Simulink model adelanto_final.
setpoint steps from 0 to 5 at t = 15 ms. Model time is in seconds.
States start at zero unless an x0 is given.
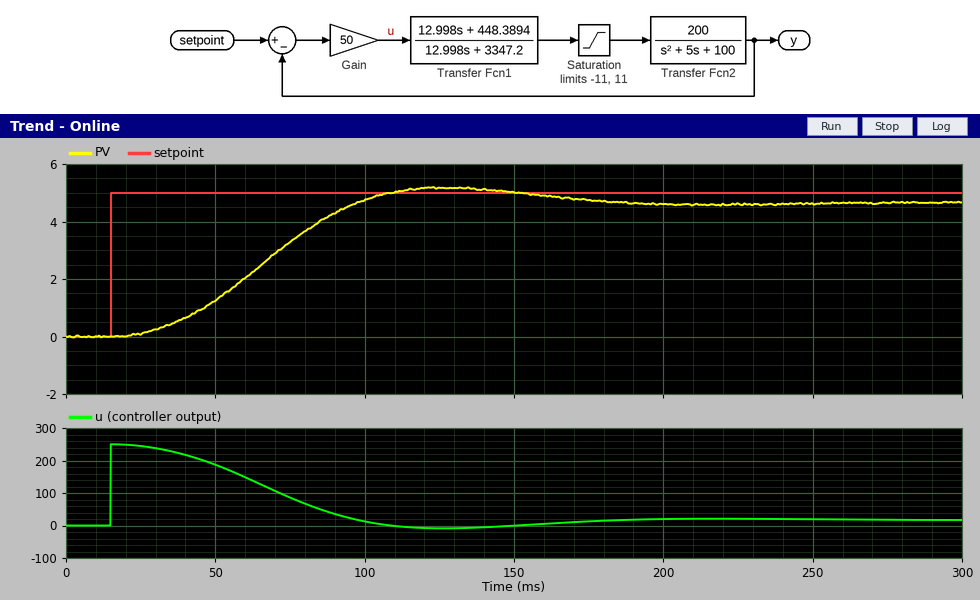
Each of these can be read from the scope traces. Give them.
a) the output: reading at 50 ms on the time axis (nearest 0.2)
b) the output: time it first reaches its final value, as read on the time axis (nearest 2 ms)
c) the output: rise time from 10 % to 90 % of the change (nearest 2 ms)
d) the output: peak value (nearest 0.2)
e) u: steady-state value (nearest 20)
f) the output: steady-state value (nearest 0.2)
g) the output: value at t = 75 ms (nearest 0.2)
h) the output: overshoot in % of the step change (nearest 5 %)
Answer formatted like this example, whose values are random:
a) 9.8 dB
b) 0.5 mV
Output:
a) 1.2
b) 98 ms
c) 52 ms
d) 5.2
e) 20
f) 4.6
g) 3.2
h) 10 %
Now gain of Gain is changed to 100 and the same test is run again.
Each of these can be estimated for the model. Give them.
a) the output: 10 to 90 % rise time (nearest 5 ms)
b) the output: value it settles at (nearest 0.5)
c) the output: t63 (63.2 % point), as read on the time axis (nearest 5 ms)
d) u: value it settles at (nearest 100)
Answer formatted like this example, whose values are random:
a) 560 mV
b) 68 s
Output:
a) 55 ms
b) 5.0
c) 70 ms
d) 0
